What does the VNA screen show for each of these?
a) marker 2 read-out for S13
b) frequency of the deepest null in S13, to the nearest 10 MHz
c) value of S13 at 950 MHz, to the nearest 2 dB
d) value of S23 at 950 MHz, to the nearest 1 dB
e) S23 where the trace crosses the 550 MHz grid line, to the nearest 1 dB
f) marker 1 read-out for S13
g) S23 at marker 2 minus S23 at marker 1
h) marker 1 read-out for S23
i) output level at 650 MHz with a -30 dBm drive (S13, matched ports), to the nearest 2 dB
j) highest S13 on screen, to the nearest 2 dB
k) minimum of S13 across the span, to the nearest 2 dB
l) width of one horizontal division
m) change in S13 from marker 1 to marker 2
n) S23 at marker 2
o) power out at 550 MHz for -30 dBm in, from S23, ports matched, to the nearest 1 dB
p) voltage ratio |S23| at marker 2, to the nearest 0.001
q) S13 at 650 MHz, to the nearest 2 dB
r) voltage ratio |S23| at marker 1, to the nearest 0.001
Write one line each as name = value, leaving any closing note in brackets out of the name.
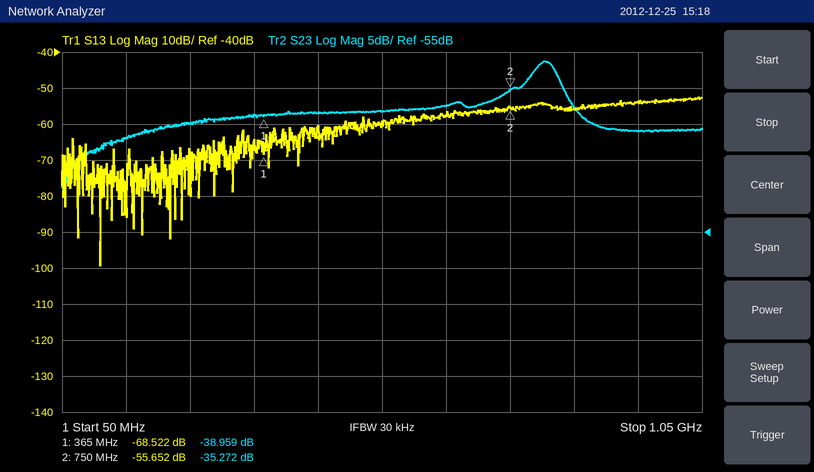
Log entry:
marker 2 read-out for S13 = -55.652 dB
frequency of the deepest null in S13, to the nearest 10 MHz = 110 MHz
value of S13 at 950 MHz, to the nearest 2 dB = -54 dB
value of S23 at 950 MHz, to the nearest 1 dB = -41 dB
S23 where the trace crosses the 550 MHz grid line, to the nearest 1 dB = -38 dB
marker 1 read-out for S13 = -68.522 dB
S23 at marker 2 minus S23 at marker 1 = 3.687 dB
marker 1 read-out for S23 = -38.959 dB
output level at 650 MHz with a -30 dBm drive (S13, matched ports), to the nearest 2 dB = -88 dBm
highest S13 on screen, to the nearest 2 dB = -52 dB
minimum of S13 across the span, to the nearest 2 dB = -100 dB
width of one horizontal division = 100 MHz
change in S13 from marker 1 to marker 2 = 12.870 dB
S23 at marker 2 = -35.272 dB
power out at 550 MHz for -30 dBm in, from S23, ports matched, to the nearest 1 dB = -68 dBm
voltage ratio |S23| at marker 2, to the nearest 0.001 = 0.017
S13 at 650 MHz, to the nearest 2 dB = -58 dB
voltage ratio |S23| at marker 1, to the nearest 0.001 = 0.011
